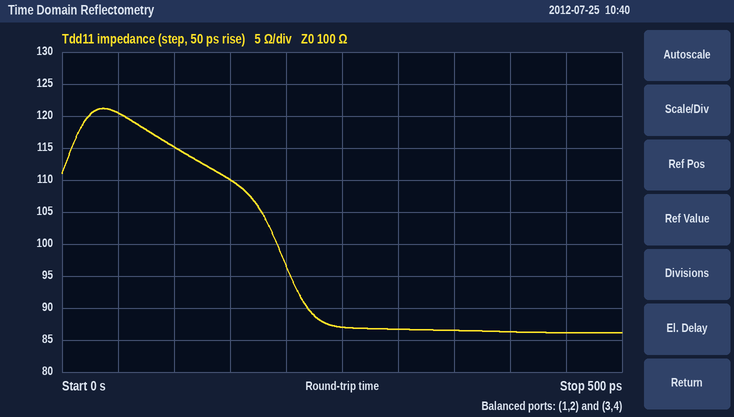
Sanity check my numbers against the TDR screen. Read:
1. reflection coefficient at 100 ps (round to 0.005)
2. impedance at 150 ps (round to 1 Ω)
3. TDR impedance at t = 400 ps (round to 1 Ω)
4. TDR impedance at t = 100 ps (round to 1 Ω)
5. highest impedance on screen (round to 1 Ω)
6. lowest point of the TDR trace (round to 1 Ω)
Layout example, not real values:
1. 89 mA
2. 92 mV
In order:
1. +0.070
2. 110 Ω
3. 86 Ω
4. 115 Ω
5. 121 Ω
6. 86 Ω
